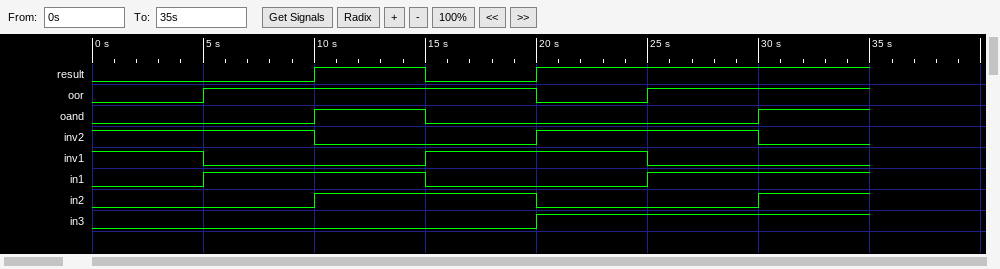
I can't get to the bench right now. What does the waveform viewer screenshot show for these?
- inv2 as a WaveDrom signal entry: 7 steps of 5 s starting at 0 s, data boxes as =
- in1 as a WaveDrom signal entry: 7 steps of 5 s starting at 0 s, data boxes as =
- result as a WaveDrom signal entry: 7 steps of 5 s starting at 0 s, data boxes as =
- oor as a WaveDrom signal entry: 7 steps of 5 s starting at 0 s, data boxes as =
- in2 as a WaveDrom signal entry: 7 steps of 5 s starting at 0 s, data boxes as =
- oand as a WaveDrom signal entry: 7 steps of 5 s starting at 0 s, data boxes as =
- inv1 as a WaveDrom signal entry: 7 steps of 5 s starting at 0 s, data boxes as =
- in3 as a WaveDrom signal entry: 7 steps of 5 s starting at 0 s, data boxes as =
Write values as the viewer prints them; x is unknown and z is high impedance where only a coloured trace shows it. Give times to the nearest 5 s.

{name: 'inv2', wave: '1.0.1.0'}
{name: 'in1', wave: '01.0.1.'}
{name: 'result', wave: '0.101..'}
{name: 'oor', wave: '01..01.'}
{name: 'in2', wave: '0.1.0.1'}
{name: 'oand', wave: '0.10..1'}
{name: 'inv1', wave: '10.1.0.'}
{name: 'in3', wave: '0...1..'}
